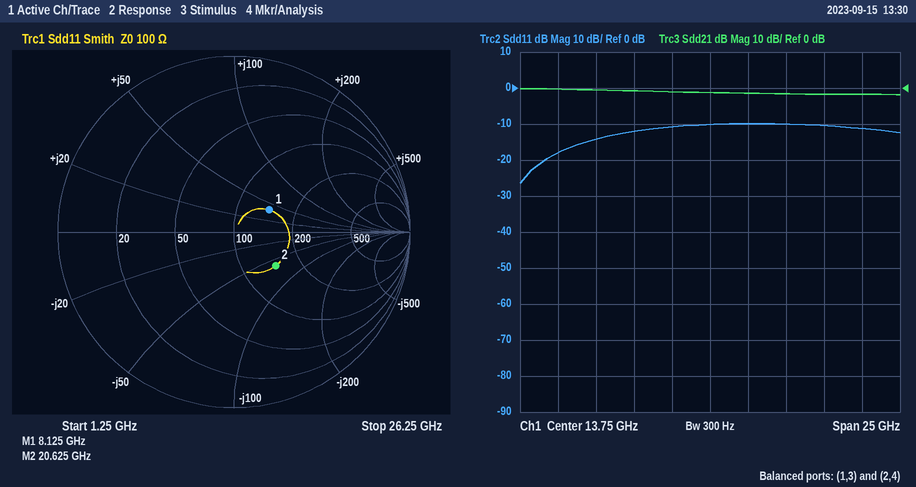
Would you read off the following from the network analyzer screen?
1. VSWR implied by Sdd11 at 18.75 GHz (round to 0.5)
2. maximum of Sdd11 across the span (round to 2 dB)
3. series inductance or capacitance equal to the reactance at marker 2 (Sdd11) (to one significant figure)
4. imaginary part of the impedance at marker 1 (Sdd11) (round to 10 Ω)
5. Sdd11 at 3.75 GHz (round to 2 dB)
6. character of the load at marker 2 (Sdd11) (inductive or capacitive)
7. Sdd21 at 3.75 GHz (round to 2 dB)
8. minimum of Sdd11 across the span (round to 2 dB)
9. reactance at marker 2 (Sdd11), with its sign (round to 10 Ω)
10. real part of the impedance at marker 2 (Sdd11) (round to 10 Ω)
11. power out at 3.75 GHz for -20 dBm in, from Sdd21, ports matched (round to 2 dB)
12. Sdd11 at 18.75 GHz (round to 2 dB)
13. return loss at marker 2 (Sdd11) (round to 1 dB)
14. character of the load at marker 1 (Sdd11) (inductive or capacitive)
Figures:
2.0
-10 dB
100 fF
+40 Ω
-18 dB
capacitive
0 dB
-26 dB
-60 Ω
150 Ω
-20 dBm
-10 dB
10 dB
inductive
